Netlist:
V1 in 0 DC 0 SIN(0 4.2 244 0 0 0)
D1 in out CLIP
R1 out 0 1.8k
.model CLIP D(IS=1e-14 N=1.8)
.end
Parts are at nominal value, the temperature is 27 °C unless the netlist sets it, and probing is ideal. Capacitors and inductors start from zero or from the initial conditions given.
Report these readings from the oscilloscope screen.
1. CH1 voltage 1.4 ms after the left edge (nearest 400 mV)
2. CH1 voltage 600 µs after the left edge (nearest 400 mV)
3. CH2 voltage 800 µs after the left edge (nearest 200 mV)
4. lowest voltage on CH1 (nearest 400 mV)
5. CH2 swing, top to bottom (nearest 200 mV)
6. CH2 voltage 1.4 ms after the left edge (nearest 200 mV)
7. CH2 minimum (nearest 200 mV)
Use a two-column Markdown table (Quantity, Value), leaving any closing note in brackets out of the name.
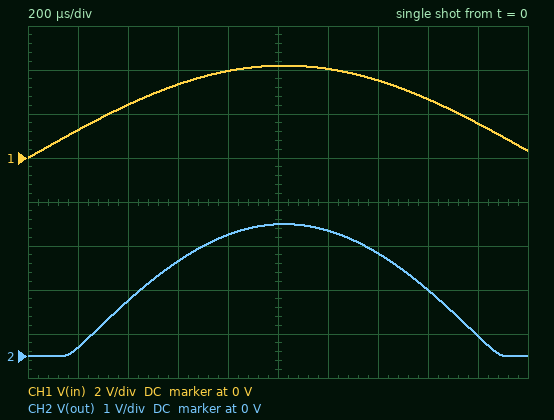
| Quantity | Value |
|---|---|
| CH1 voltage 1.4 ms after the left edge | 3.6 V |
| CH1 voltage 600 µs after the left edge | 3.2 V |
| CH2 voltage 800 µs after the left edge | 2.8 V |
| lowest voltage on CH1 | 0 V |
| CH2 swing, top to bottom | 3.0 V |
| CH2 voltage 1.4 ms after the left edge | 2.4 V |
| CH2 minimum | 0 V |
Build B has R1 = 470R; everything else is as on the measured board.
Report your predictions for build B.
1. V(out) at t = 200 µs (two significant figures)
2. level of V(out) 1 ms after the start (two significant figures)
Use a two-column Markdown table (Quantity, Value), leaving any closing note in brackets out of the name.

| Quantity | Value |
|---|---|
| V(out) at t = 200 µs | 140 mV |
| level of V(out) 1 ms after the start | 2.9 V |
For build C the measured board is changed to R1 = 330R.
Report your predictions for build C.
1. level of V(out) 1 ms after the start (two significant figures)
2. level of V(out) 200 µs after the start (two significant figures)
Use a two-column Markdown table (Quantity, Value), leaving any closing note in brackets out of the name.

| Quantity | Value |
|---|---|
| level of V(out) 1 ms after the start | 2.9 V |
| level of V(out) 200 µs after the start | 130 mV |
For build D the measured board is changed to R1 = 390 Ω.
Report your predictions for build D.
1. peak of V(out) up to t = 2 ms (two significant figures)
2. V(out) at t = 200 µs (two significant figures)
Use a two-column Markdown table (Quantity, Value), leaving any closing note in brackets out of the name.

| Quantity | Value |
|---|---|
| peak of V(out) up to t = 2 ms | 2.9 V |
| V(out) at t = 200 µs | 140 mV |
